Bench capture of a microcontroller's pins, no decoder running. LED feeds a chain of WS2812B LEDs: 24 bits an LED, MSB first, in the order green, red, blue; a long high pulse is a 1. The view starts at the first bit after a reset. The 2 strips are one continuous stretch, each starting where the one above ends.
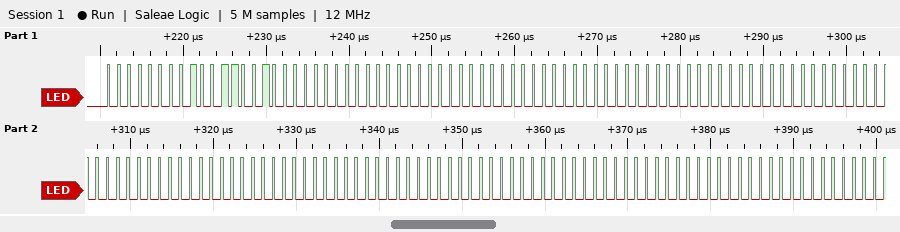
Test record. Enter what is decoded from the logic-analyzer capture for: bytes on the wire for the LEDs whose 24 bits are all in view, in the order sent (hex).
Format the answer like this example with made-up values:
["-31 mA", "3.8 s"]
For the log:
["00 99 00 00 00 00 00 00 00 00 00 00 00 00 00 00 00 00"]
